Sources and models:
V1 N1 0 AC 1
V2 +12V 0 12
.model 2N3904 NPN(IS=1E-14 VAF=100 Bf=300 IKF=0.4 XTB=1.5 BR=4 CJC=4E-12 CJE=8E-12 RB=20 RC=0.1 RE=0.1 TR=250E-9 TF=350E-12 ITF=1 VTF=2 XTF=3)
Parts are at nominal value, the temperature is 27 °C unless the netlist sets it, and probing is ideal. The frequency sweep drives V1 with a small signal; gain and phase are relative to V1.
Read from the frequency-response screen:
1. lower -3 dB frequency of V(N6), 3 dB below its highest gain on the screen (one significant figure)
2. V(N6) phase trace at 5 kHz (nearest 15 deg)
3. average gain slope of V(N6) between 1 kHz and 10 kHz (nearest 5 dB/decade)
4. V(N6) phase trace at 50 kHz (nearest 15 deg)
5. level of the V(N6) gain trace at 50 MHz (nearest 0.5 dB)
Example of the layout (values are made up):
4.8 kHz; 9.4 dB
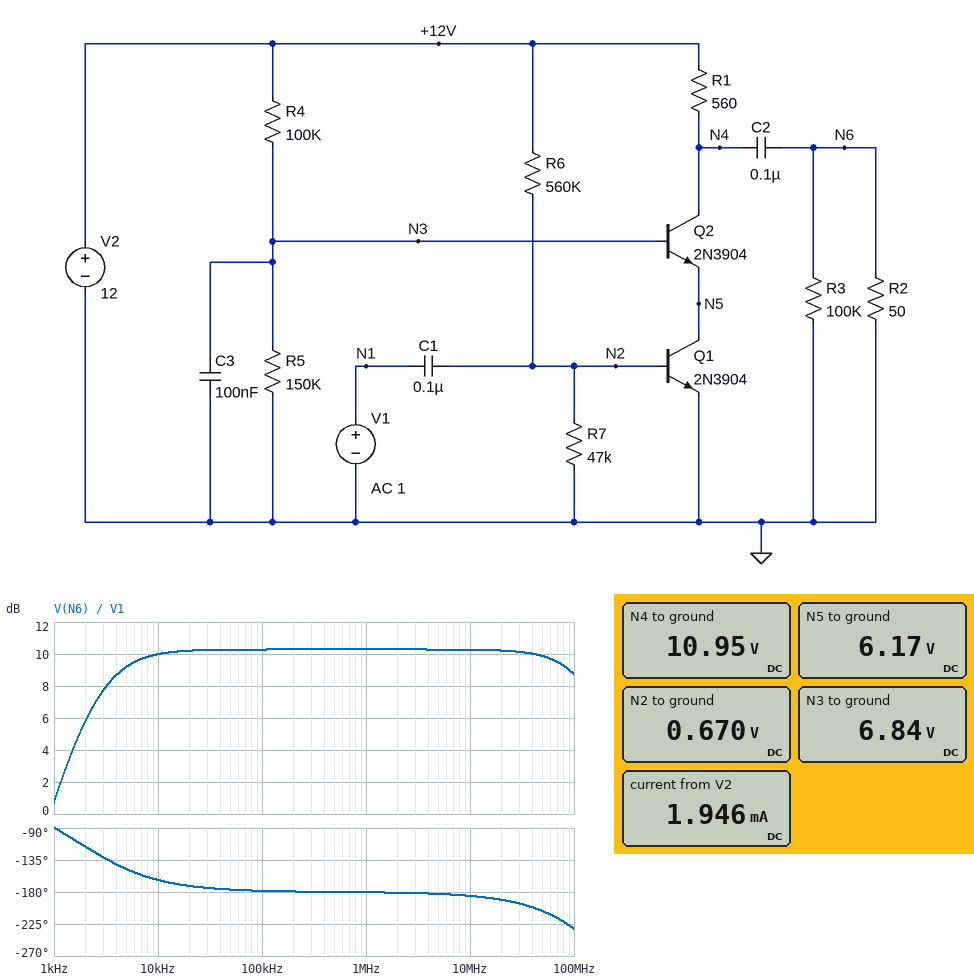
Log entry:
3 kHz; -150 deg; 10 dB/decade; -180 deg; 10.0 dB
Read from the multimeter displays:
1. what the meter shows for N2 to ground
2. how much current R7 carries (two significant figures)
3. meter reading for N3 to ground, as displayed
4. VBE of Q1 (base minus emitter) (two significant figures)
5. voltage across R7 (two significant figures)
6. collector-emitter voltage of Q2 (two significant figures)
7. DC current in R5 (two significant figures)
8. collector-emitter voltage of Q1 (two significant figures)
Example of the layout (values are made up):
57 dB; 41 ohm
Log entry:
0.670 V; 14 µA; 6.84 V; 670 mV; 670 mV; 4.8 V; 46 µA; 6.2 V
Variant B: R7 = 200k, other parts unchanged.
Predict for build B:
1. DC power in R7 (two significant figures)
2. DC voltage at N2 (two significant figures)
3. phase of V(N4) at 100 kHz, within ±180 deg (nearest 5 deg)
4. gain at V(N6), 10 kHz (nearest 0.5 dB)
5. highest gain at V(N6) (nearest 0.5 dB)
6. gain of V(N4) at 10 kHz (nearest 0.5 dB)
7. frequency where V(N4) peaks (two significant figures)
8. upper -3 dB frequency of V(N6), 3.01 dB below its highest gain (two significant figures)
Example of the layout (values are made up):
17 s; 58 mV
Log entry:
2.4 µW; 700 mV; 165 deg; 18.5 dB; 19.0 dB; 29.0 dB; 1.6 kHz; 90 MHz
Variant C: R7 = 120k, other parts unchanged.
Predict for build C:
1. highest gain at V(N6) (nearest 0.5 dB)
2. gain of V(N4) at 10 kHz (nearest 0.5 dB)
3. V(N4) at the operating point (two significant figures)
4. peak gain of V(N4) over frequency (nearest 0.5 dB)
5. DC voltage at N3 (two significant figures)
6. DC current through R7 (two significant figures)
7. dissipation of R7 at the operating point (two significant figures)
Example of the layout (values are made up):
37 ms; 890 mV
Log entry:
17.5 dB; 28.0 dB; 9.5 V; 37.0 dB; 6.3 V; 5.8 µA; 4.0 µW
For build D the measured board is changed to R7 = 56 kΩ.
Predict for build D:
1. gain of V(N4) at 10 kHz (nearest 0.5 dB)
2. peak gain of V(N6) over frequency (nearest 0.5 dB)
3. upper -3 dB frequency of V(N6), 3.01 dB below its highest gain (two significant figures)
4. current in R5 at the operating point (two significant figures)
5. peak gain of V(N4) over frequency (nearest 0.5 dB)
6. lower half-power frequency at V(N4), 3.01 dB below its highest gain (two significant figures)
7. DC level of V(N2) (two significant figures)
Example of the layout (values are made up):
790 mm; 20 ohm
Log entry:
23.0 dB; 13.0 dB; 130 MHz; 45 µA; 33.0 dB; 390 Hz; 680 mV
